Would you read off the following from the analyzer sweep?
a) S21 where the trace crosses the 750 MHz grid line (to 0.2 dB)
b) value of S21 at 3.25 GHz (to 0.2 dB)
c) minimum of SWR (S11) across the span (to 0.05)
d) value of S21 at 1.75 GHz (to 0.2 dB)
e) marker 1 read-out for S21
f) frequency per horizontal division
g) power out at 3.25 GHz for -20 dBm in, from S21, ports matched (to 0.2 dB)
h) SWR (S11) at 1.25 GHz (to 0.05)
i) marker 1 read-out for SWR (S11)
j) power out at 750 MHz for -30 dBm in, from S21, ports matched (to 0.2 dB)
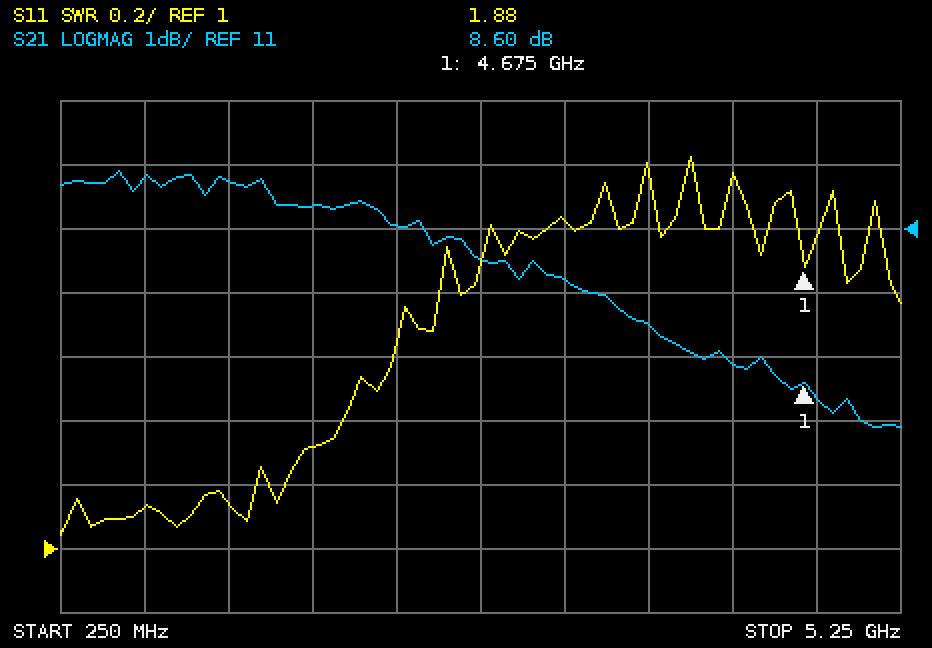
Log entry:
11.8 dB
10.2 dB
1.05
11.4 dB
8.60 dB
500 MHz
-9.8 dBm
1.15
1.88
-18.2 dBm
